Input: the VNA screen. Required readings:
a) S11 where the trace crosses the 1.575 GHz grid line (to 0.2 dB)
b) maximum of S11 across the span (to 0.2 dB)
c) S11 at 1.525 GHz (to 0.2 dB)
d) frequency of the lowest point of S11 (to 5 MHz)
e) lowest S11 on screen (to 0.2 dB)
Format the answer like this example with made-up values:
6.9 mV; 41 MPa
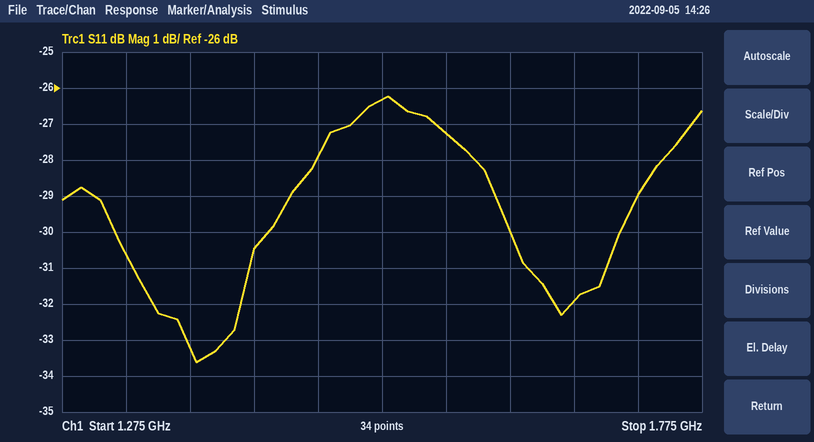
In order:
-27.2 dB; -26.2 dB; -26.4 dB; 1.380 GHz; -33.6 dB
